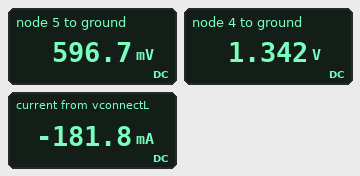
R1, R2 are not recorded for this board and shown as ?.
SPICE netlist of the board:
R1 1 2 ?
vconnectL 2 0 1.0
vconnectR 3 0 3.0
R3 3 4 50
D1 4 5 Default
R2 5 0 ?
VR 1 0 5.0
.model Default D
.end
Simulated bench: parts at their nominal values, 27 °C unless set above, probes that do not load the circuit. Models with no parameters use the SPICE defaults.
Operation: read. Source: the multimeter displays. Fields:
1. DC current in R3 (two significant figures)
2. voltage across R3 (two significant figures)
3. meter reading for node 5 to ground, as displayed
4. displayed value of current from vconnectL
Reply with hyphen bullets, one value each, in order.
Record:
- 33 mA
- 1.7 V
- 596.7 mV
- -181.8 mA
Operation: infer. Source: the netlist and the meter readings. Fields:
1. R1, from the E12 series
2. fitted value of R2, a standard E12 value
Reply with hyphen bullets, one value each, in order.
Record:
- 22 Ω
- 18 Ω
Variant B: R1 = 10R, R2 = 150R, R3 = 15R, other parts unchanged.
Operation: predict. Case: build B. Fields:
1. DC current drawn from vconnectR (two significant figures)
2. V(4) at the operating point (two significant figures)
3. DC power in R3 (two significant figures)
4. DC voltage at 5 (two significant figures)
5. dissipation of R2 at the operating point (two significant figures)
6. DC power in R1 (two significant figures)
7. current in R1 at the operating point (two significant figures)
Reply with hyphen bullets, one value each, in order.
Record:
- 14 mA
- 2.8 V
- 2.9 mW
- 2.1 V
- 29 mW
- 1.6 W
- 400 mA
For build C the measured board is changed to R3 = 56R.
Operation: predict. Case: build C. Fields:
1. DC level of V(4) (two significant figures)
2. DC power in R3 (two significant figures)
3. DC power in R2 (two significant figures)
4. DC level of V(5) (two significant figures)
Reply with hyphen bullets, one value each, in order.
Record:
- 1.3 V
- 52 mW
- 17 mW
- 550 mV
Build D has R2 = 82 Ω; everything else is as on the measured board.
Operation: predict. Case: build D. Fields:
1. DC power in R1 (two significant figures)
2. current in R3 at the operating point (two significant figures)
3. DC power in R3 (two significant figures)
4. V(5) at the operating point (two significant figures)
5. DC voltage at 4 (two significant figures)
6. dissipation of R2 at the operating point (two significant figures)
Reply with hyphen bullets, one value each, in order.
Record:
- 730 mW
- 17 mA
- 15 mW
- 1.4 V
- 2.1 V
- 24 mW
